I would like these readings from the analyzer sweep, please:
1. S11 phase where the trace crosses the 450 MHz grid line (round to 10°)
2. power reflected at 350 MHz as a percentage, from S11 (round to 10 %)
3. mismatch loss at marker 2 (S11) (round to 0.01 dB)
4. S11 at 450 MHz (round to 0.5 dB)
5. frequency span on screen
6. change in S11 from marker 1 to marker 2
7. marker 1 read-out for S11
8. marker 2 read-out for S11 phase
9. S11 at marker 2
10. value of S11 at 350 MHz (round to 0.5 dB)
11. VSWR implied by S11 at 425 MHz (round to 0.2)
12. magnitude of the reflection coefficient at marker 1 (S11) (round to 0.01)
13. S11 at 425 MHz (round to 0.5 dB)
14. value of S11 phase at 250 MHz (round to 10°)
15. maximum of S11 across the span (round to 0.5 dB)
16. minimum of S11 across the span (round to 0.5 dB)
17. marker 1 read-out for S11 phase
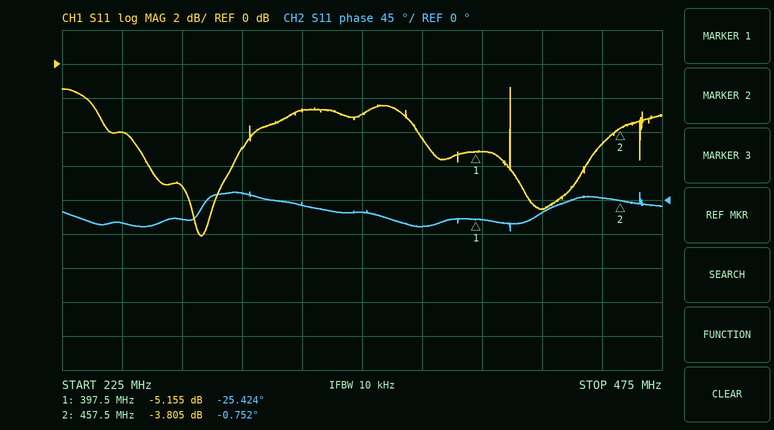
0°
50 %
2.34 dB
-4.5 dB
250 MHz
1.350 dB
-5.155 dB
-0.752°
-3.805 dB
-3.0 dB
2.2
0.55
-8.5 dB
-30°
-1.5 dB
-10.0 dB
-25.424°
